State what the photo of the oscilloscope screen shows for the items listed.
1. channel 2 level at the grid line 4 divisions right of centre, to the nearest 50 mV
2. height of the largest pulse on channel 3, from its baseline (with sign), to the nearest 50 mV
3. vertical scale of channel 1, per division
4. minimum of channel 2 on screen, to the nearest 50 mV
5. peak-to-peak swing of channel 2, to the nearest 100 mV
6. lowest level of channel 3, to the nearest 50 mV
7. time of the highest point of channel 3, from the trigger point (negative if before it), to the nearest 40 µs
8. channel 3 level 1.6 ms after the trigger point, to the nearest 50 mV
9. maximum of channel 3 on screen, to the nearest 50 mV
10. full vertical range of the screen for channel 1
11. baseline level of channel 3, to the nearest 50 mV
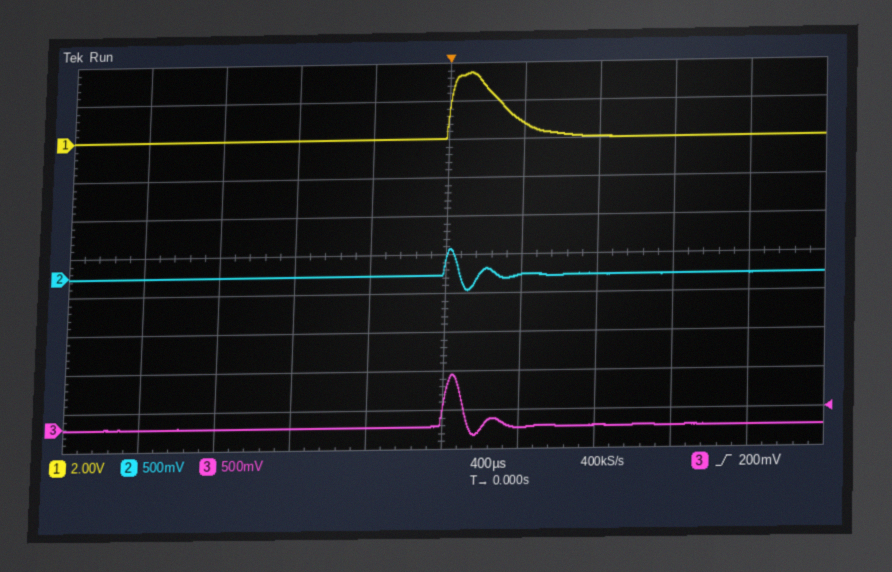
0 mV
+650 mV
2 V
-200 mV
500 mV
-100 mV
+40 µs
0 mV
650 mV
20 V
0 mV
